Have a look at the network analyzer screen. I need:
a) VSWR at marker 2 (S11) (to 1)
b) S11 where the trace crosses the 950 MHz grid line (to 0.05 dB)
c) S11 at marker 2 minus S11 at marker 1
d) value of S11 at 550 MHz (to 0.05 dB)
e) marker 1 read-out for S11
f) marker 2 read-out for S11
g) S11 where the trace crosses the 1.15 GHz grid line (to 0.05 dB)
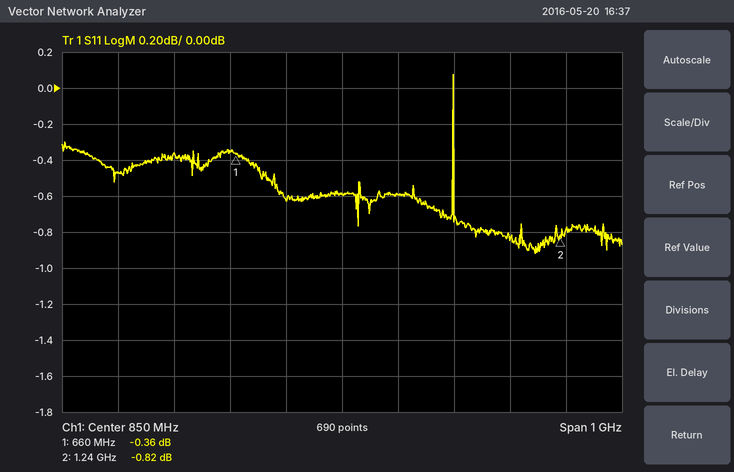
21
-0.60 dB
-0.46 dB
-0.35 dB
-0.36 dB
-0.82 dB
-0.85 dB
